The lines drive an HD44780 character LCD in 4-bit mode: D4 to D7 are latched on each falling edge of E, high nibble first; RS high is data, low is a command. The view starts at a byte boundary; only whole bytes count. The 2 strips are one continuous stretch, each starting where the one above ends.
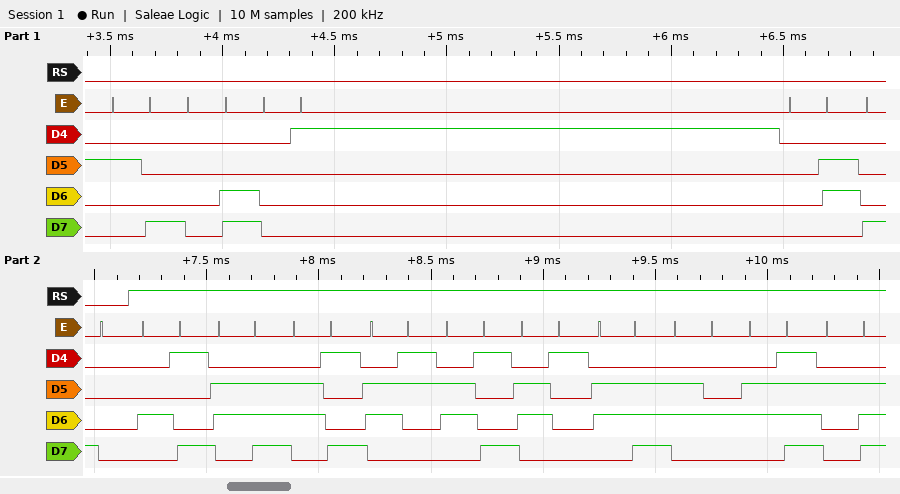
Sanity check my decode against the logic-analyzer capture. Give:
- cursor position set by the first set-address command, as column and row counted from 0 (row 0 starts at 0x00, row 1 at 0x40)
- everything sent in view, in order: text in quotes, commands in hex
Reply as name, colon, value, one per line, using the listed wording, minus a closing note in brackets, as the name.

cursor position set by the first set-address command, as column and row counted from 0: column 0, row 0
everything sent in view, in order: text in quotes, commands in hex: 0x28 0x0C 0x01 0x06 0x80 "Iniciando."
